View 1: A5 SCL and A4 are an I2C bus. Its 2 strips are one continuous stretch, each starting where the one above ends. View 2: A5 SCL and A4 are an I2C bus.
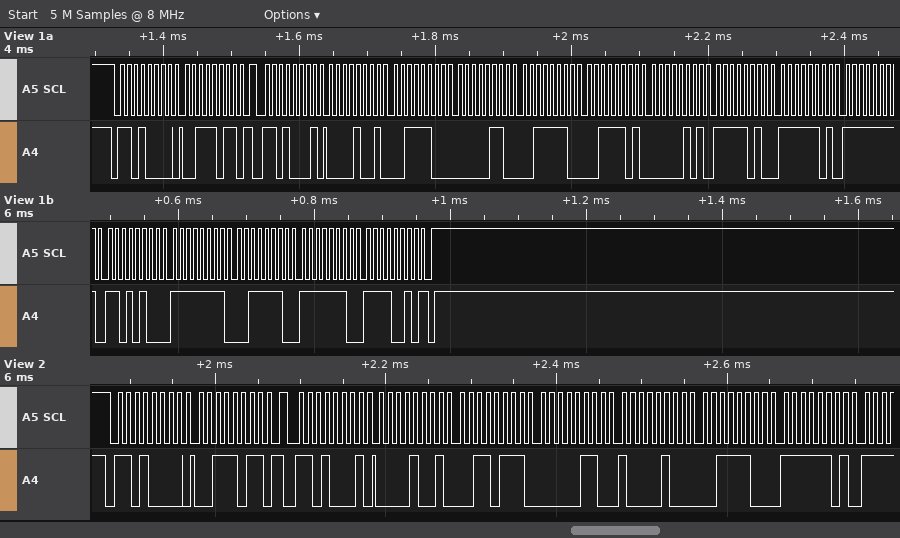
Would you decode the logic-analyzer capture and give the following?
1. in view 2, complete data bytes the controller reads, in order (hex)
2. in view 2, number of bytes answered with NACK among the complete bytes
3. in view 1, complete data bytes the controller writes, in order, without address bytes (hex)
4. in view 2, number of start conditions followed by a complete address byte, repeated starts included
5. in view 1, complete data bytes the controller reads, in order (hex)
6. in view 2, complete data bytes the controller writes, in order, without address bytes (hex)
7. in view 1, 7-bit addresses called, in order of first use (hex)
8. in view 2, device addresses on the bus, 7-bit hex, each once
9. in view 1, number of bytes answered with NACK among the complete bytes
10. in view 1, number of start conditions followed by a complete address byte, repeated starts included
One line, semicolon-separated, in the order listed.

09 37 06 84 3C FD; 0; 3B; 2; 09 3C 06 3E 3D 05 FA FD FF D4 FF 3E FE F2; 3B; 0x68; 0x68; 1; 2
